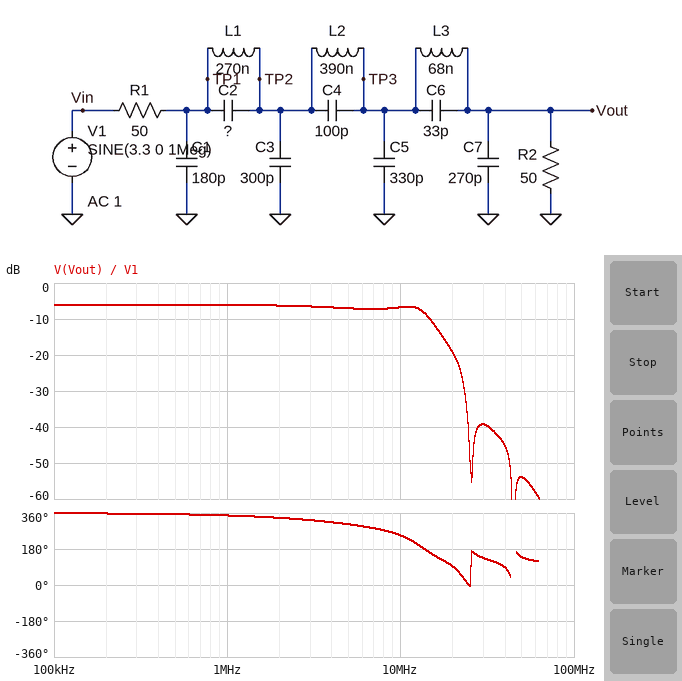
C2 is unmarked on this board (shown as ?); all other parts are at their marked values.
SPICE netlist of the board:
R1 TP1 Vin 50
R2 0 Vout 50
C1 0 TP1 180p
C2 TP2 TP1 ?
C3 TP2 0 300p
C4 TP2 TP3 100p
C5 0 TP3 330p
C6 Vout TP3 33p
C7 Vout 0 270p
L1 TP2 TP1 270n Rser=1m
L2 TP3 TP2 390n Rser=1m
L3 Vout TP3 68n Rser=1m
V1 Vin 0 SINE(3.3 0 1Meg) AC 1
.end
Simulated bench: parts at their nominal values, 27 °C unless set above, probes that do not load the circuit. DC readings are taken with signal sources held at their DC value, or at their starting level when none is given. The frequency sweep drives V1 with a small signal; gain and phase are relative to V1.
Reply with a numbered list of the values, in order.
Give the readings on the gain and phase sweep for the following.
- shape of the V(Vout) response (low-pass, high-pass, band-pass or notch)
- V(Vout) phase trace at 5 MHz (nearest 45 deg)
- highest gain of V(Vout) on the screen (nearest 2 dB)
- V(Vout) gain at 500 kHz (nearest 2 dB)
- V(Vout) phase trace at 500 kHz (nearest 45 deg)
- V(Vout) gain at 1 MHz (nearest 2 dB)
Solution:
1. low-pass
2. 315 deg
3. -6 dB
4. -6 dB
5. 360 deg
6. -6 dB
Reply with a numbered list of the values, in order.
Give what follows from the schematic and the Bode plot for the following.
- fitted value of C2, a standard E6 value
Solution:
1. 47 pF
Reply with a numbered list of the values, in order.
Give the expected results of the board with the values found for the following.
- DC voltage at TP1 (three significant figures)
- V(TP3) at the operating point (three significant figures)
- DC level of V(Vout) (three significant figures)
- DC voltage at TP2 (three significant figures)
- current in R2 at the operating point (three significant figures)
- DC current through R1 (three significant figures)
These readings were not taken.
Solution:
1. 1.65 V
2. 1.65 V
3. 1.65 V
4. 1.65 V
5. 33.0 mA
6. 33.0 mA
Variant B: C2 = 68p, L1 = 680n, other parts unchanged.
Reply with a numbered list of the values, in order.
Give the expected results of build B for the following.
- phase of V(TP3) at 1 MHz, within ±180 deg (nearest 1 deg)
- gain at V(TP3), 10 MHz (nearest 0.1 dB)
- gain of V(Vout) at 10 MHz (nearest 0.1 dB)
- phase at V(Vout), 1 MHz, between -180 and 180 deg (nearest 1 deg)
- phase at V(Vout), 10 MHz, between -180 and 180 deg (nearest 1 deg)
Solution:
1. -13 deg
2. -9.0 dB
3. -8.4 dB
4. -14 deg
5. -143 deg
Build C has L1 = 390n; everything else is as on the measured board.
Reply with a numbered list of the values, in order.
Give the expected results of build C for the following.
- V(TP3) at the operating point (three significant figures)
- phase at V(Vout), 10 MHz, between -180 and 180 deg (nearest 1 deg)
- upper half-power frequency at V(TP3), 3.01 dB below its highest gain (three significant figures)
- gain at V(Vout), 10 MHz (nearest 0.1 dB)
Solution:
1. 1.65 V
2. -121 deg
3. 13.0 MHz
4. -6.9 dB
